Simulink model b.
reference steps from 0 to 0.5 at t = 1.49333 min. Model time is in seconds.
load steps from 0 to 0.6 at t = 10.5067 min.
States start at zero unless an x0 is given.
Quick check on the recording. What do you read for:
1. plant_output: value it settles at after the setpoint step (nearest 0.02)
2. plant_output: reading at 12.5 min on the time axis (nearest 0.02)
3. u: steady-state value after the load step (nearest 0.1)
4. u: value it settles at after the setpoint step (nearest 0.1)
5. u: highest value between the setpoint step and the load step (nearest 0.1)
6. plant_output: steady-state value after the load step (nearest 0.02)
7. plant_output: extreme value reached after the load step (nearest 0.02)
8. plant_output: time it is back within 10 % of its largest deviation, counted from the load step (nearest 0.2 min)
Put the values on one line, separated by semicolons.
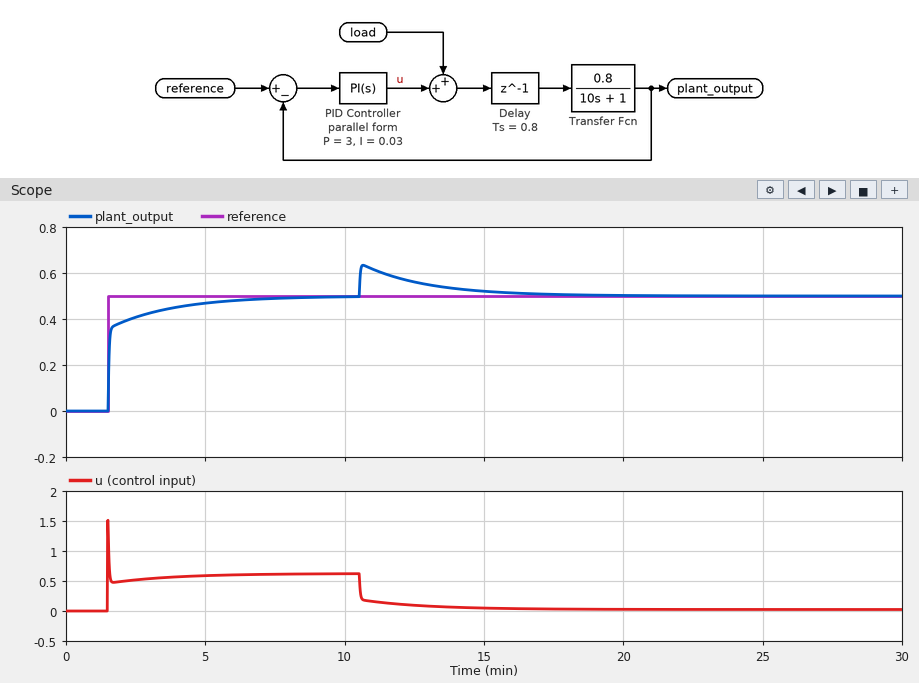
0.50; 0.56; 0.0; 0.6; 1.5; 0.50; 0.64; 5.4 min
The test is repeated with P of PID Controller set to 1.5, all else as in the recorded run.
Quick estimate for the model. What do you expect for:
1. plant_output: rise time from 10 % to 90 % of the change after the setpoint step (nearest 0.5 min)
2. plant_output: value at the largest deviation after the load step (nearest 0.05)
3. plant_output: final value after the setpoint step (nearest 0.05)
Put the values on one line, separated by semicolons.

2.0 min; 0.70; 0.50
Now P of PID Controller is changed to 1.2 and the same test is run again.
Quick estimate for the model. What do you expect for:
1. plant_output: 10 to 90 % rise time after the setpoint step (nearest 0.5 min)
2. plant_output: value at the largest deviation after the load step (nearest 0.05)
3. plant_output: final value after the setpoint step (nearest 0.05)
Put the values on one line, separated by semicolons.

2.0 min; 0.70; 0.50
